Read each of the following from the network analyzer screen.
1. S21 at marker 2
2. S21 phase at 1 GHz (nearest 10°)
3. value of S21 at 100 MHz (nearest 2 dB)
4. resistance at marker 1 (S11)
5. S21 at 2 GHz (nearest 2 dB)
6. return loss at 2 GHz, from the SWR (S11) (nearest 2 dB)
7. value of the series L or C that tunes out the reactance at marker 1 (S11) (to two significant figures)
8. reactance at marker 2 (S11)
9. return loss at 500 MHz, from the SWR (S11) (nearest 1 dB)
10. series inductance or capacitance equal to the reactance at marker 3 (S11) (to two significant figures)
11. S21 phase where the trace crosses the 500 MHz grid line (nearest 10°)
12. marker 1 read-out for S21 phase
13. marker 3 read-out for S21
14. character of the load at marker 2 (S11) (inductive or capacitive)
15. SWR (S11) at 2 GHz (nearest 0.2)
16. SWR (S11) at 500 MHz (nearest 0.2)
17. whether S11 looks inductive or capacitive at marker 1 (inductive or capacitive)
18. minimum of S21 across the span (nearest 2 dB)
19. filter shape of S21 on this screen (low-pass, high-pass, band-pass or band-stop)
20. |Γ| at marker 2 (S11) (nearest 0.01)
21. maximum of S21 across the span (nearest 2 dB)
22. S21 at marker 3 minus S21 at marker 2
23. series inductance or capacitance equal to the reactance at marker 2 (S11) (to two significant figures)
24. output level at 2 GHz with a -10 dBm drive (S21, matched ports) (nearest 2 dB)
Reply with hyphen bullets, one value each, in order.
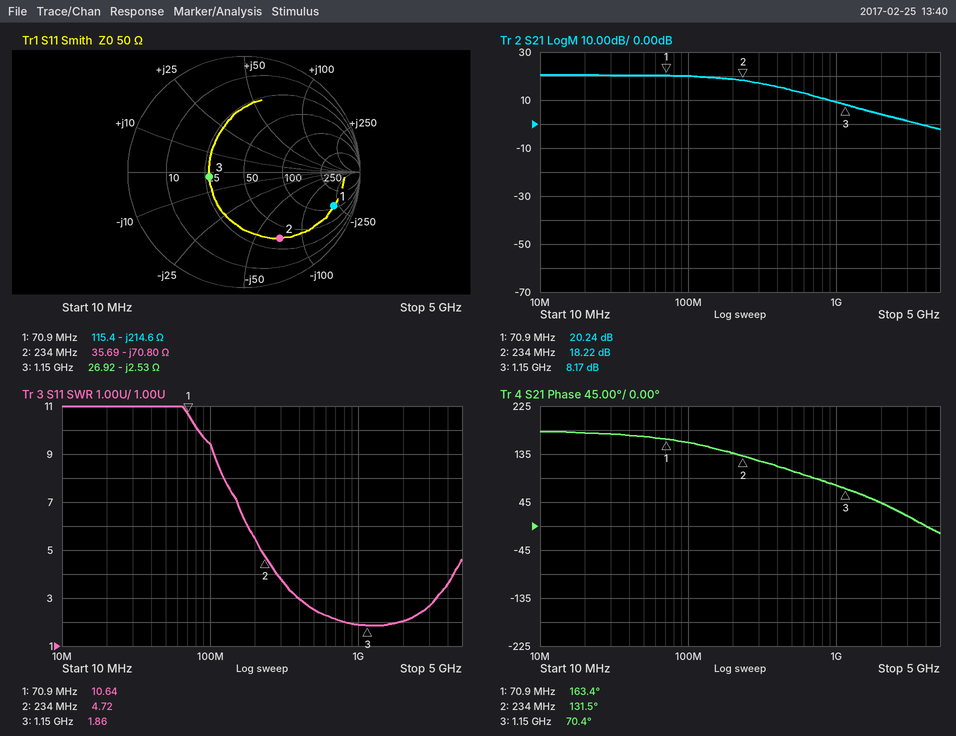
- 18.22 dB
- 80°
- 20 dB
- 115.4 Ω
- 4 dB
- 10 dB
- 480 nH
- -70.80 Ω
- 7 dB
- 55 pF
- 100°
- 163.4°
- 8.17 dB
- capacitive
- 2.0
- 2.6
- capacitive
- -2 dB
- low-pass
- 0.65
- 20 dB
- -10.05 dB
- 9.6 pF
- -6 dBm
